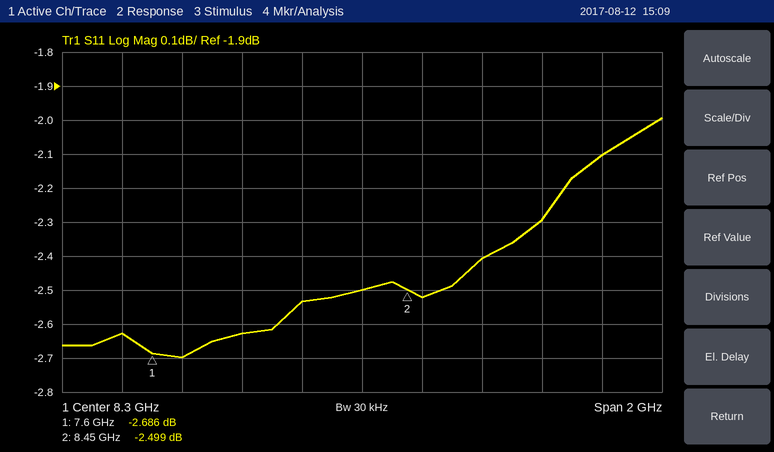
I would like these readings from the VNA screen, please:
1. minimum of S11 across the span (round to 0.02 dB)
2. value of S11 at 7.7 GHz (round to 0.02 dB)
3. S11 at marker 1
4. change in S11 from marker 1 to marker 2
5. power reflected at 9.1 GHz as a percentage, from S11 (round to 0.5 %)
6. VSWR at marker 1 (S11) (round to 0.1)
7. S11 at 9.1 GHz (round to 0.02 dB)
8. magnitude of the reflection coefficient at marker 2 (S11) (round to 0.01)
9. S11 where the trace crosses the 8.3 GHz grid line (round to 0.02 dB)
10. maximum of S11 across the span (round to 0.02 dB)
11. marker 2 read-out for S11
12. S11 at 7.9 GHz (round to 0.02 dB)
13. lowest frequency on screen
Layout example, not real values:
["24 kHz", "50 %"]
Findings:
["-2.70 dB", "-2.70 dB", "-2.686 dB", "0.187 dB", "61.5 %", "6.5", "-2.10 dB", "0.75", "-2.50 dB", "-2.00 dB", "-2.499 dB", "-2.62 dB", "7.3 GHz"]
